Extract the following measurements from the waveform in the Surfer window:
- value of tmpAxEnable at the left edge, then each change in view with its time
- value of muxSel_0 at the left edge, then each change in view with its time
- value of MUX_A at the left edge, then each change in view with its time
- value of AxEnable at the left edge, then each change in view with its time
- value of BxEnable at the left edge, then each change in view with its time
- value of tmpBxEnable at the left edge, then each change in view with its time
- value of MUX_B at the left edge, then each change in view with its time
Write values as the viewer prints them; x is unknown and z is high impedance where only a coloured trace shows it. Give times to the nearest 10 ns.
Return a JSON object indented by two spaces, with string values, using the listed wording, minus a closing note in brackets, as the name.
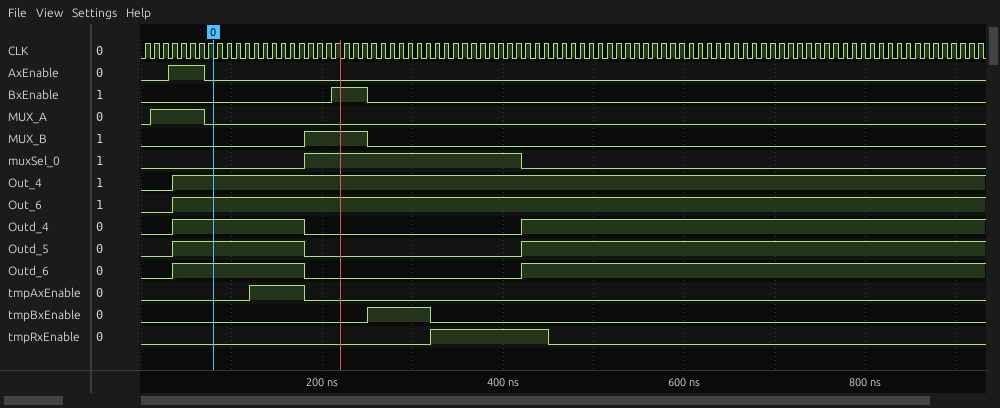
{
  "value of tmpAxEnable at the left edge, then each change in view with its time": "0, 1 at 120 ns, 0 at 180 ns",
  "value of muxSel_0 at the left edge, then each change in view with its time": "0, 1 at 180 ns, 0 at 420 ns",
  "value of MUX_A at the left edge, then each change in view with its time": "0, 1 at 10 ns, 0 at 70 ns",
  "value of AxEnable at the left edge, then each change in view with its time": "0, 1 at 30 ns, 0 at 70 ns",
  "value of BxEnable at the left edge, then each change in view with its time": "0, 1 at 210 ns, 0 at 250 ns",
  "value of tmpBxEnable at the left edge, then each change in view with its time": "0, 1 at 250 ns, 0 at 320 ns",
  "value of MUX_B at the left edge, then each change in view with its time": "0, 1 at 180 ns, 0 at 250 ns"
}
